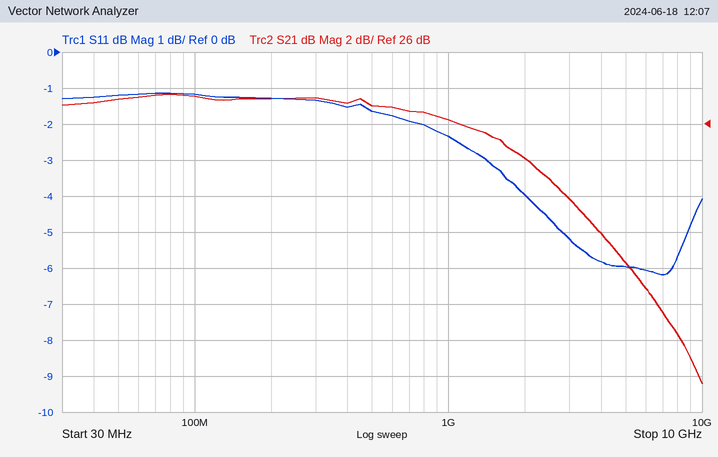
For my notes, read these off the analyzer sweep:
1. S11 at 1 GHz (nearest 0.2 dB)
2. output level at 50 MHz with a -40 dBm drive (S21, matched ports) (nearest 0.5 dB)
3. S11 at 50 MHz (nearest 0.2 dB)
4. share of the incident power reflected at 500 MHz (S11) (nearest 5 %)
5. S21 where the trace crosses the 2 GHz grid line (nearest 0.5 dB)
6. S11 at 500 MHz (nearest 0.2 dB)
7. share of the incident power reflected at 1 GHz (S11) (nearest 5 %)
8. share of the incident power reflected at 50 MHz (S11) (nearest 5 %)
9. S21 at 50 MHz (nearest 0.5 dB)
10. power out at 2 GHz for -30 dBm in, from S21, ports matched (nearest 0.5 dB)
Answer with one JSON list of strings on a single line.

["-2.4 dB", "-12.5 dBm", "-1.2 dB", "70 %", "24.0 dB", "-1.6 dB", "60 %", "75 %", "27.5 dB", "-6.0 dBm"]
